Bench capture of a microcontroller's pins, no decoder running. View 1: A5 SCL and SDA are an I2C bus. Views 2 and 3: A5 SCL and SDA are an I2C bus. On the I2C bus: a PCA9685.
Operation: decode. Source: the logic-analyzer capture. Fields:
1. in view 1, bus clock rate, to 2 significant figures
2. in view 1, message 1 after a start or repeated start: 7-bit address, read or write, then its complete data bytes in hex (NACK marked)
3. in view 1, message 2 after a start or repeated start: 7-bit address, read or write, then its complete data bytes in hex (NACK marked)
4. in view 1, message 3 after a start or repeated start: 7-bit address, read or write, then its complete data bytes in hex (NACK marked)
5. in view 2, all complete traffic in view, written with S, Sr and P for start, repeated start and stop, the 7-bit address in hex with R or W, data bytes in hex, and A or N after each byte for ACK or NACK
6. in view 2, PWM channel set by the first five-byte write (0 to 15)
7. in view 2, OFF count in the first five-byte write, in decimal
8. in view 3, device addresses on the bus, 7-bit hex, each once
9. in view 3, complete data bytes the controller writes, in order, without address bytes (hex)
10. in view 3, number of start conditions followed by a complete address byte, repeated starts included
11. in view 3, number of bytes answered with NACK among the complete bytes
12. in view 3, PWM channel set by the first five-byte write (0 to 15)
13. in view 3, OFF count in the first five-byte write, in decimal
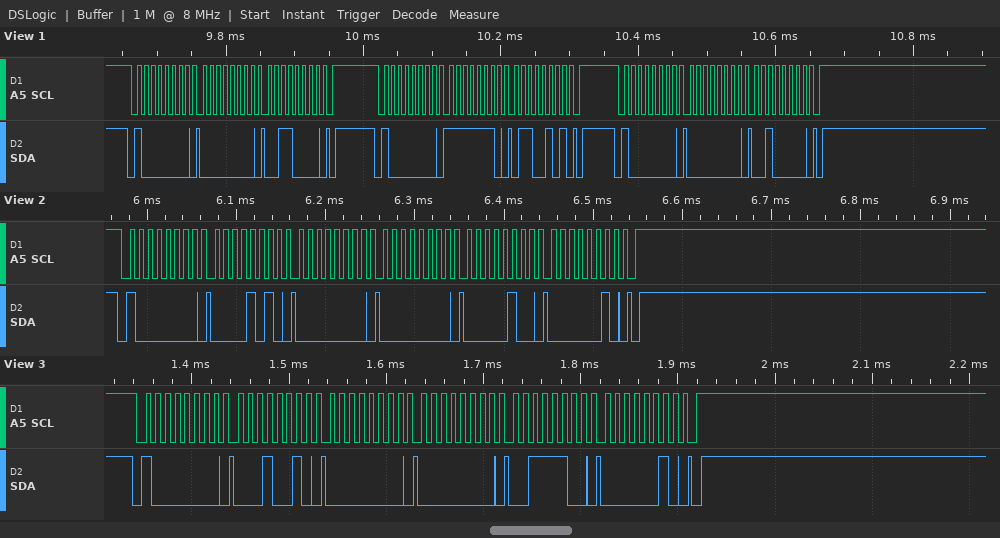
100 kHz
0x40 write: 00 30
0x40 write: FE 65
0x40 write: 00 20
S 40W A 0A A 00 A 00 A 04 A 02 A P
1
516
0x40
12 00 00 3C 02
1
0
3
572
